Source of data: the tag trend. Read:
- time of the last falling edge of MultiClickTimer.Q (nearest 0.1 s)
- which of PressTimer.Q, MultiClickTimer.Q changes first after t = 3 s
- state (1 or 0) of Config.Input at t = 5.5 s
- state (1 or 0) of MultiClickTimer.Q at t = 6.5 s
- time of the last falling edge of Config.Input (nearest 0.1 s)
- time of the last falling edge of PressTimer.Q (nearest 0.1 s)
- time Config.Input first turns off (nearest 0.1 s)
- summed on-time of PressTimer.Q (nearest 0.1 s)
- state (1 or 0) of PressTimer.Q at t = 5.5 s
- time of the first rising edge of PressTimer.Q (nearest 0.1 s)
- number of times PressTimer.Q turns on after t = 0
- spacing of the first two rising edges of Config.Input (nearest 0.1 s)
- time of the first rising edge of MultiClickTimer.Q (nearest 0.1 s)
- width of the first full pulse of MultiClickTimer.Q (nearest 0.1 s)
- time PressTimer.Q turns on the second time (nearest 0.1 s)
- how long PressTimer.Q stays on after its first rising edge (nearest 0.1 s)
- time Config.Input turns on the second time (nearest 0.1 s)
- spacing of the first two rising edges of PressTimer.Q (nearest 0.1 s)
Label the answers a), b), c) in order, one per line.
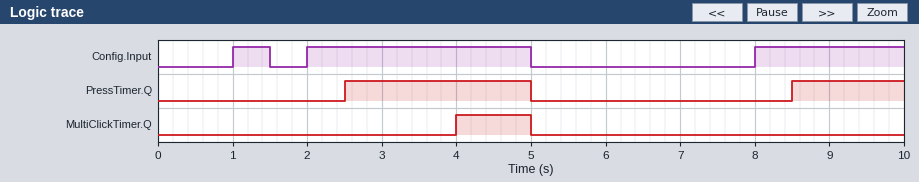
a) 5.0 s
b) MultiClickTimer.Q
c) 0
d) 0
e) 5.0 s
f) 5.0 s
g) 1.5 s
h) 4.0 s
i) 0
j) 2.5 s
k) 2
l) 1.0 s
m) 4.0 s
n) 1.0 s
o) 8.5 s
p) 2.5 s
q) 2.0 s
r) 6.0 s
